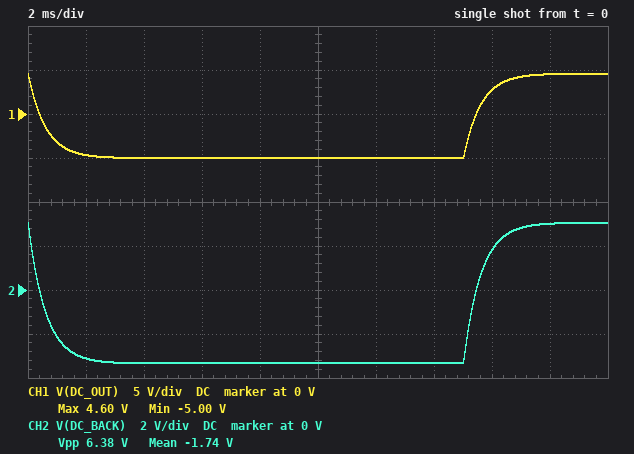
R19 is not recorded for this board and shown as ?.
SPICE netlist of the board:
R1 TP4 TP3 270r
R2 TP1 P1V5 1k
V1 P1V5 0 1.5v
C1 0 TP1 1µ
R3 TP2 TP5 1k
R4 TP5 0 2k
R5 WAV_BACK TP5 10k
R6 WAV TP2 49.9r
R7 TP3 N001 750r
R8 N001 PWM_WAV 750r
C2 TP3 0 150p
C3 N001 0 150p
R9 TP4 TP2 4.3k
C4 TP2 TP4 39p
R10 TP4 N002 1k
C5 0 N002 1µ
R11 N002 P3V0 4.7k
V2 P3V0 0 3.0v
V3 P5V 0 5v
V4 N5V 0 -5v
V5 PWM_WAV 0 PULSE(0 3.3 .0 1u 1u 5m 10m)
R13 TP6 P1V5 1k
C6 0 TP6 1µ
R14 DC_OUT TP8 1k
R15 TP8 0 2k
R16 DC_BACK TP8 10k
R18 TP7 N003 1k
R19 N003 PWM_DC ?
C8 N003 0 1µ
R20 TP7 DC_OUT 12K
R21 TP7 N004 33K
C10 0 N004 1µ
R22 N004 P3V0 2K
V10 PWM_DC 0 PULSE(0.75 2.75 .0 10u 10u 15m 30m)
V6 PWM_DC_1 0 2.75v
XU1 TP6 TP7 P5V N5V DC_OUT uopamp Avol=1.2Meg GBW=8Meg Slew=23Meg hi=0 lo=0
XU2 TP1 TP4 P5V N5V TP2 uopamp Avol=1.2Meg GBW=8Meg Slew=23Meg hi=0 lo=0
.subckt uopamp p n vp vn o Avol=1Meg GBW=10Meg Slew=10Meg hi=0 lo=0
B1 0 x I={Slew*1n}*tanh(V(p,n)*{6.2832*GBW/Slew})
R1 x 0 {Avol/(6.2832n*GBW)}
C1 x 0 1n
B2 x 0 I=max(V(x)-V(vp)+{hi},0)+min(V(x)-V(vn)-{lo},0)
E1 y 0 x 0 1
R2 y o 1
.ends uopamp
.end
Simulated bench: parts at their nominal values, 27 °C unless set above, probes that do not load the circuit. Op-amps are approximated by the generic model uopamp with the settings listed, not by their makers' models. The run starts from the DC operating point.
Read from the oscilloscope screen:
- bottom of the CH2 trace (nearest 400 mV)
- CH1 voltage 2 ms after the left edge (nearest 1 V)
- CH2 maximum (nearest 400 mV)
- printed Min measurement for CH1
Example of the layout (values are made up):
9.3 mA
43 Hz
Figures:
-3.2 V
-5 V
3.2 V
-5.00 V
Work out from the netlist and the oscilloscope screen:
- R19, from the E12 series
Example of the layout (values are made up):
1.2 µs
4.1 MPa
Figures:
1.5 kΩ
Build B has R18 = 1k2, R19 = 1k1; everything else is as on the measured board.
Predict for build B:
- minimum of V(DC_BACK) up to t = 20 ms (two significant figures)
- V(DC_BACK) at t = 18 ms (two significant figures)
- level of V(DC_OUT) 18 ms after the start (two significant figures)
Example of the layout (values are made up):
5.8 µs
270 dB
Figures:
-3.3 V
3.2 V
4.8 V
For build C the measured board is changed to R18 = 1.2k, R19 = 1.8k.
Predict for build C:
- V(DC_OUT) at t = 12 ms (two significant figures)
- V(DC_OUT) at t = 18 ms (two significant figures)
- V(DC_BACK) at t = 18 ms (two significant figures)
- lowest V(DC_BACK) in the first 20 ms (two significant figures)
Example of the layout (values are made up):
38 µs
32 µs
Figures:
-4.0 V
3.9 V
2.6 V
-2.7 V
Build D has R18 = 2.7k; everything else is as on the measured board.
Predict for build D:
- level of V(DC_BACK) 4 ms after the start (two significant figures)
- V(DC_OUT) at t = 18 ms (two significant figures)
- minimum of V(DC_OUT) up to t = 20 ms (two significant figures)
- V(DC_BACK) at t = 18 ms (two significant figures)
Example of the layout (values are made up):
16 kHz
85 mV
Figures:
-1.7 V
2.9 V
-2.6 V
1.9 V
